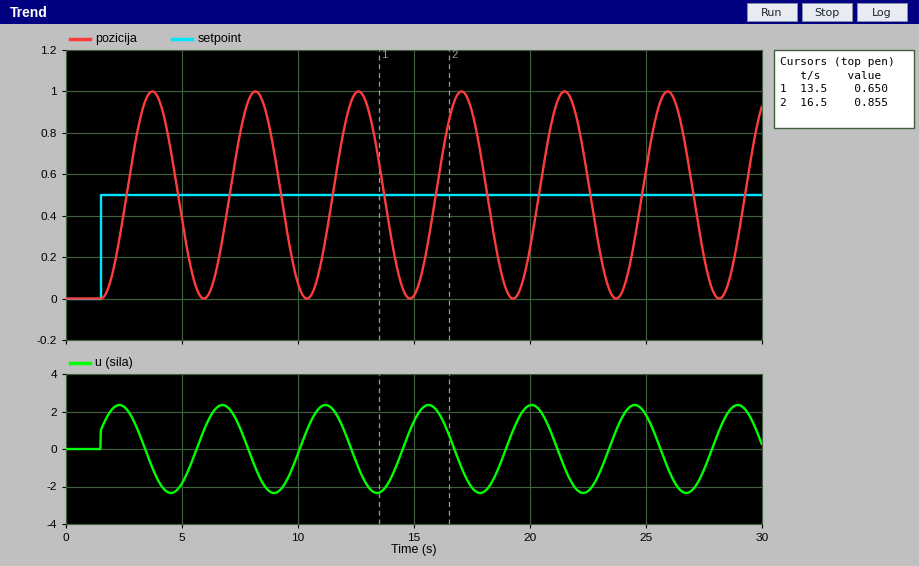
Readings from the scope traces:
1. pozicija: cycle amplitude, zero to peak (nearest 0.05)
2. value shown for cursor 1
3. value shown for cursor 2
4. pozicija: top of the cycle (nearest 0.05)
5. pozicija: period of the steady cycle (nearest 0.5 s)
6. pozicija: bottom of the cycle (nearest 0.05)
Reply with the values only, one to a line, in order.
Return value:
0.50
0.650
0.855
1.00
4.5 s
0.00
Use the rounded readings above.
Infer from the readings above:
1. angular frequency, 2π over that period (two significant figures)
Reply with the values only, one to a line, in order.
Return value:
1.4 rad/s
